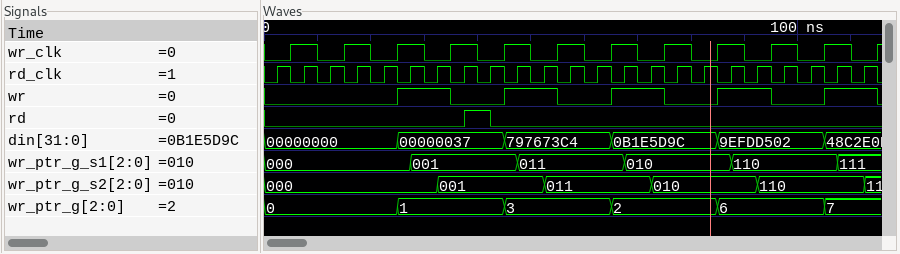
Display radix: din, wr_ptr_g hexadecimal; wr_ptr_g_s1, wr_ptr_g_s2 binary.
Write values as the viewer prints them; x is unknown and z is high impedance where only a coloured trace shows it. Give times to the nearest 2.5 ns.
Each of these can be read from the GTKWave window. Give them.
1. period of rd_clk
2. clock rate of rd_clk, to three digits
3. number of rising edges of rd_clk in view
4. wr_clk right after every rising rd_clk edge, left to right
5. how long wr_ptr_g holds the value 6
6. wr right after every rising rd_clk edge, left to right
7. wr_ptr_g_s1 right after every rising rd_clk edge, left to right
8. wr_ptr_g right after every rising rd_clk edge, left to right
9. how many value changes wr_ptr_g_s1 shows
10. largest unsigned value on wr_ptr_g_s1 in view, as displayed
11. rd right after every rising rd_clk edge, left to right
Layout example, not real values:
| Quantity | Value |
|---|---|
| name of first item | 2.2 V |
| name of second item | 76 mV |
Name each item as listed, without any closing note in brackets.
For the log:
| Quantity | Value |
|---|---|
| period of rd_clk | 5 ns |
| clock rate of rd_clk, to three digits | 200 MHz |
| number of rising edges of rd_clk in view | 23 |
| wr_clk right after every rising rd_clk edge, left to right | 0 1 0 1 0 1 0 1 0 1 0 1 0 1 0 1 0 1 0 1 0 1 0 |
| how long wr_ptr_g holds the value 6 | 20 ns |
| wr right after every rising rd_clk edge, left to right | 0 0 0 0 0 1 1 0 0 1 1 0 0 1 1 0 0 1 1 0 0 1 1 |
| wr_ptr_g_s1 right after every rising rd_clk edge, left to right | 000, 000, 000, 000, 000, 001, 001, 001, 001, 011, 011, 011, 011, 010, 010, 010, 010, 110, 110, 110, 110, 111, 111 |
| wr_ptr_g right after every rising rd_clk edge, left to right | 0, 0, 0, 0, 0, 1, 1, 1, 1, 3, 3, 3, 3, 2, 2, 2, 2, 6, 6, 6, 6, 7, 7 |
| how many value changes wr_ptr_g_s1 shows | 5 |
| largest unsigned value on wr_ptr_g_s1 in view, as displayed | 111 |
| rd right after every rising rd_clk edge, left to right | 0 0 0 0 0 0 0 1 0 0 0 0 0 0 0 0 0 0 0 0 0 0 0 |
